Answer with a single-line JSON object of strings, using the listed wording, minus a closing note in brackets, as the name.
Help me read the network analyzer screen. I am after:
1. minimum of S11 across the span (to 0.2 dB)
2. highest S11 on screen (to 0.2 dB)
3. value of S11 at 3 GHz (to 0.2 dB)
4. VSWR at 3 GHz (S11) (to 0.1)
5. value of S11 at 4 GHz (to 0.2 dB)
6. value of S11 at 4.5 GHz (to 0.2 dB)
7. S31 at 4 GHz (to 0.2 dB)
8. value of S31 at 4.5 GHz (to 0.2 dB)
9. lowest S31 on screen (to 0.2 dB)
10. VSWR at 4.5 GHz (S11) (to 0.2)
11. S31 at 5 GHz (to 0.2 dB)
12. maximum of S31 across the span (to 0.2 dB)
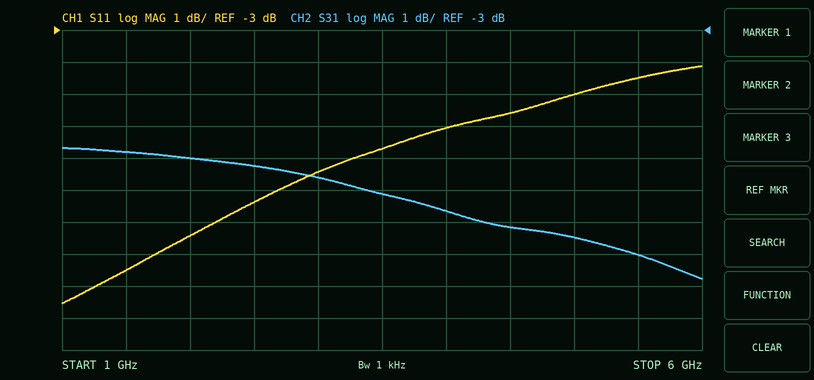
{"minimum of S11 across the span": "-11.6 dB", "highest S11 on screen": "-4.2 dB", "value of S11 at 3 GHz": "-7.4 dB", "VSWR at 3 GHz (S11)": "2.5", "value of S11 at 4 GHz": "-6.0 dB", "value of S11 at 4.5 GHz": "-5.6 dB", "S31 at 4 GHz": "-8.6 dB", "value of S31 at 4.5 GHz": "-9.2 dB", "lowest S31 on screen": "-10.8 dB", "VSWR at 4.5 GHz (S11)": "3.2", "S31 at 5 GHz": "-9.4 dB", "maximum of S31 across the span": "-6.6 dB"}
